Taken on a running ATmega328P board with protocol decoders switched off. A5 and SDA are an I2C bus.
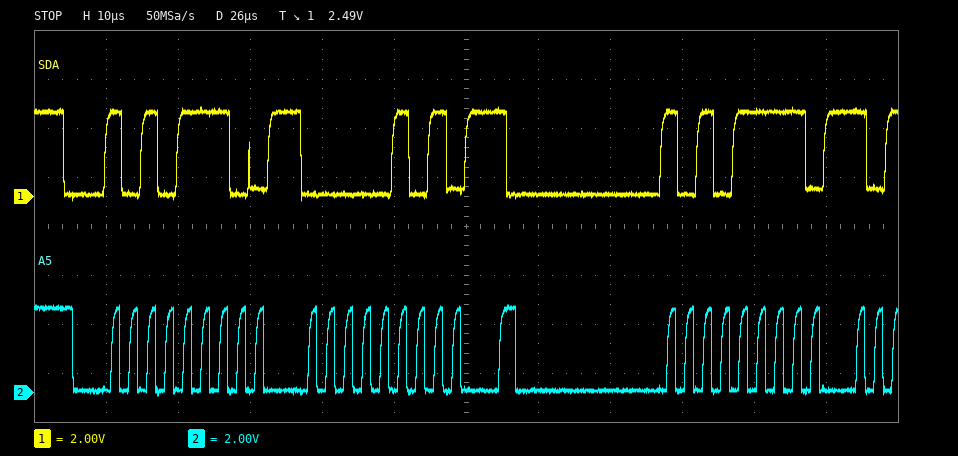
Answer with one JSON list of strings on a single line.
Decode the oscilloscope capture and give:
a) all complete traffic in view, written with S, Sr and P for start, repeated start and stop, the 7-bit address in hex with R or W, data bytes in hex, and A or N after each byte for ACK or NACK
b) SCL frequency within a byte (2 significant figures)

["S 57W A 05 A Sr 57R A", "400 kHz"]
